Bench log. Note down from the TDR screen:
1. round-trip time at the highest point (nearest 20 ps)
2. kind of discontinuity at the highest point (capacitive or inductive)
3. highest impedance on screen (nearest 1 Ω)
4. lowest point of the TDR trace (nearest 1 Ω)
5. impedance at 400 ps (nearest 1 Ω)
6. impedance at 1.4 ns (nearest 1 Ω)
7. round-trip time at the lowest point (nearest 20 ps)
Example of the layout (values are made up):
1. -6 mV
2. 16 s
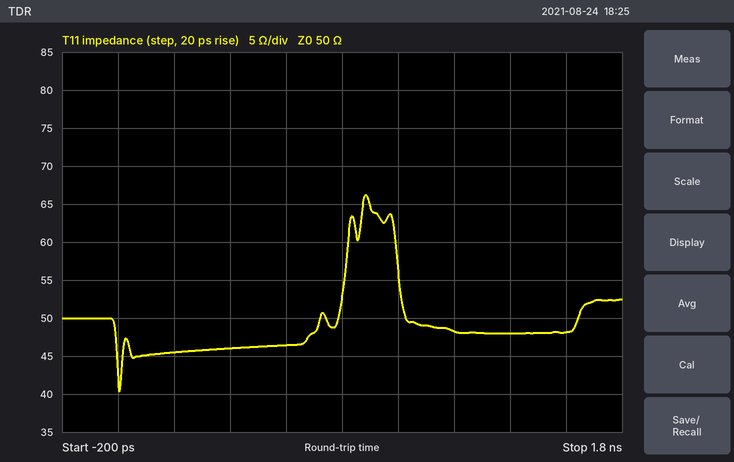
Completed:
1. 880 ps
2. inductive
3. 66 Ω
4. 40 Ω
5. 46 Ω
6. 48 Ω
7. 0 ps
